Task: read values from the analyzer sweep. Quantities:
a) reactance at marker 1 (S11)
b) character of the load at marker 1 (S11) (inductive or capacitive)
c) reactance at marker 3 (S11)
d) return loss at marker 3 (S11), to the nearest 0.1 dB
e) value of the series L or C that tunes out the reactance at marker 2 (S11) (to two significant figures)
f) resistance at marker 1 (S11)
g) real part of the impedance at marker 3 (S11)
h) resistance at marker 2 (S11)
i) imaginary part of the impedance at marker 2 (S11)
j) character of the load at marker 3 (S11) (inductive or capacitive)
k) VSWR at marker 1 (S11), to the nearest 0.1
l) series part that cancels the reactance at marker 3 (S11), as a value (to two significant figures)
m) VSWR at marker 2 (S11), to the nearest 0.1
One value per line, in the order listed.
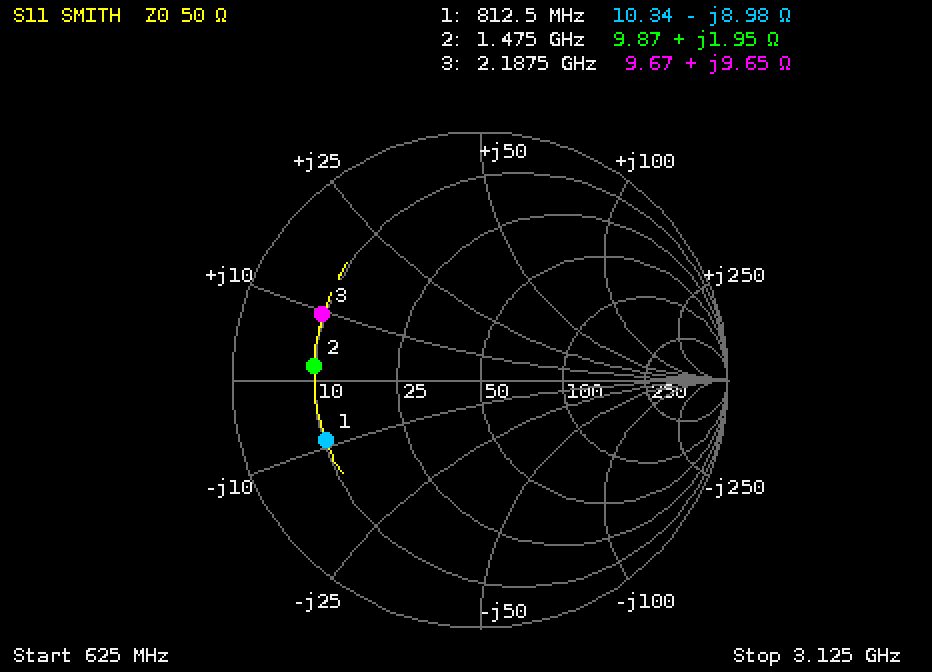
-8.98 Ω
capacitive
+9.65 Ω
3.3 dB
55 pF
10.34 Ω
9.67 Ω
9.87 Ω
+1.95 Ω
inductive
5.0
7.5 pF
5.1
